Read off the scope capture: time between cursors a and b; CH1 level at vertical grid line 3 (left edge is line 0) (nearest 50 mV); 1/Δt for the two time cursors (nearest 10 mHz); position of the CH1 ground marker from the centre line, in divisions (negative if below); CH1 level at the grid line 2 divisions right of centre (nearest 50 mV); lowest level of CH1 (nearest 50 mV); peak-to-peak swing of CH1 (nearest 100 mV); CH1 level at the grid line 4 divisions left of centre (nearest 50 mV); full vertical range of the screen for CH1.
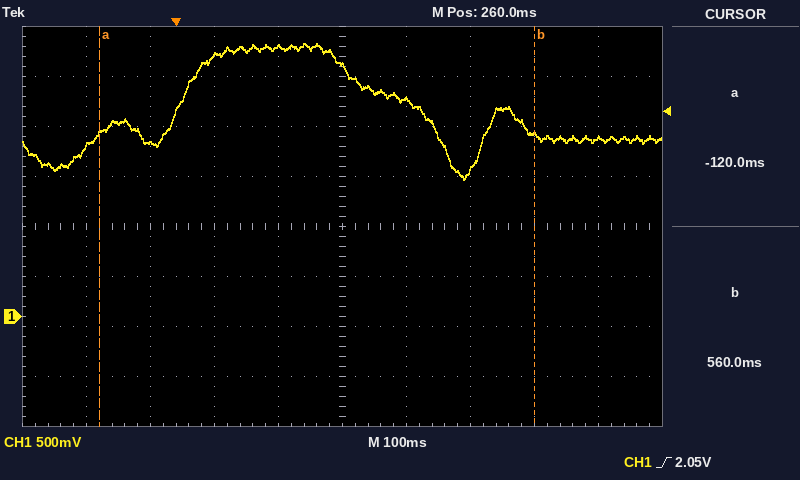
680 ms
2.60 V
1.47 Hz
-1.8 div
1.45 V
1.35 V
1.40 V
1.70 V
4 V
